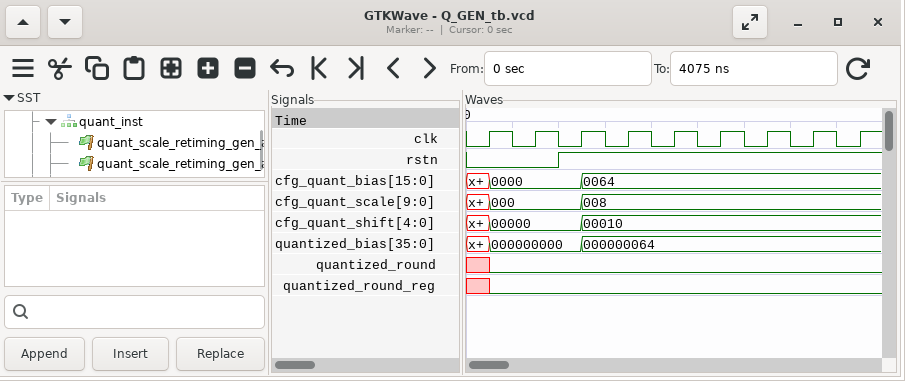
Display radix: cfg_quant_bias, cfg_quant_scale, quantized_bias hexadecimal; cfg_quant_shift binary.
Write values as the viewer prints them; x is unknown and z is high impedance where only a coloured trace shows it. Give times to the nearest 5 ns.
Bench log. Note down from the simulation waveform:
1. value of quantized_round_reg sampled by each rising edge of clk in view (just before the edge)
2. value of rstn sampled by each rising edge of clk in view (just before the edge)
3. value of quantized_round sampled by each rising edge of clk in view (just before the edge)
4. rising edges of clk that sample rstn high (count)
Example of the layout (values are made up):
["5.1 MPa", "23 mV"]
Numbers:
["x 0 0 0 0 0 0 0 0", "0 0 1 1 1 1 1 1 1", "x 0 0 0 0 0 0 0 0", "7"]
